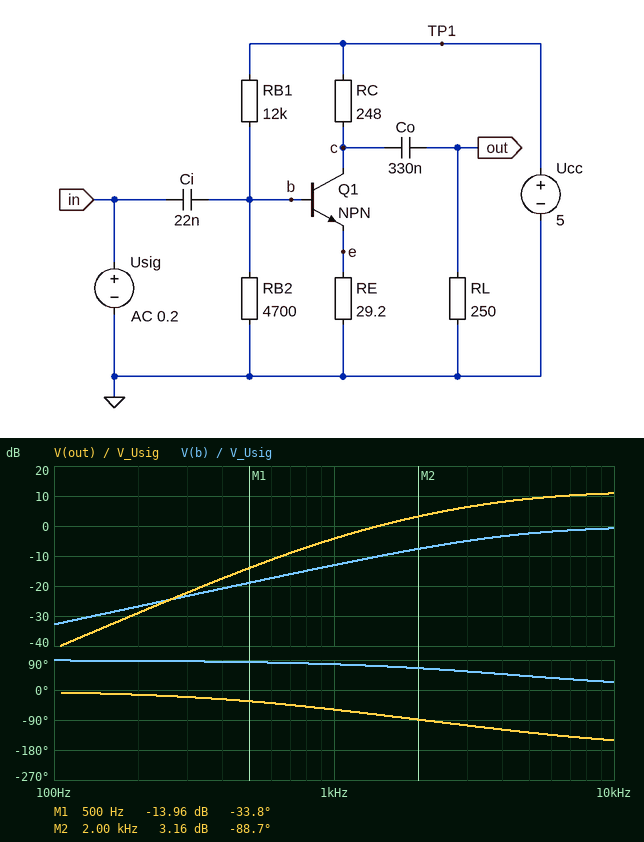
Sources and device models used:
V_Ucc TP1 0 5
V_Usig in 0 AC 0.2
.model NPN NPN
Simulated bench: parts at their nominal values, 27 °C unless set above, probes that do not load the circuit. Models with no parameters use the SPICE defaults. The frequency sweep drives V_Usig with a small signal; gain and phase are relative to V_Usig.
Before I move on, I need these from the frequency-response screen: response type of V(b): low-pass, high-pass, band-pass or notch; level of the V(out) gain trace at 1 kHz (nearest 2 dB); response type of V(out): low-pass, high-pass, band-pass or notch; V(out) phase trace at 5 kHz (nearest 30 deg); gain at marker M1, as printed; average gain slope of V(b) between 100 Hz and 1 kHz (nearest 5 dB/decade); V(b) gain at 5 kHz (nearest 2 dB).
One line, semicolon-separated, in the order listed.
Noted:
high-pass; -4 dB; high-pass; -120 deg; -13.96 dB; 20 dB/decade; -2 dB
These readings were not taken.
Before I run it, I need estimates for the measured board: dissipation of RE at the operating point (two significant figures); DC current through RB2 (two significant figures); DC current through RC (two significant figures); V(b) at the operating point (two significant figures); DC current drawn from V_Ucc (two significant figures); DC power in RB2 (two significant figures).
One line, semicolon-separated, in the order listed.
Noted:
2.5 mW; 230 µA; 9.1 mA; 1.1 V; 9.4 mA; 260 µW
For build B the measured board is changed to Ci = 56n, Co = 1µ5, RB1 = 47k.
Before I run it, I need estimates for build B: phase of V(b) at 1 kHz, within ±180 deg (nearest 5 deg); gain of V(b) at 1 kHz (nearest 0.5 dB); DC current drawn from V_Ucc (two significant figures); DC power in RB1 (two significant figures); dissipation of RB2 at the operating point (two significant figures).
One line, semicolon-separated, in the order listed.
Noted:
35 deg; -1.5 dB; 97 µA; 440 µW; 44 µW
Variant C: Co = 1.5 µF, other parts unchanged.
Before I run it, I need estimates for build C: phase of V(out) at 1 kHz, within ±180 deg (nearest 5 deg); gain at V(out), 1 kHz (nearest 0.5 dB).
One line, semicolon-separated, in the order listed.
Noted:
-90 deg; -1.5 dB
